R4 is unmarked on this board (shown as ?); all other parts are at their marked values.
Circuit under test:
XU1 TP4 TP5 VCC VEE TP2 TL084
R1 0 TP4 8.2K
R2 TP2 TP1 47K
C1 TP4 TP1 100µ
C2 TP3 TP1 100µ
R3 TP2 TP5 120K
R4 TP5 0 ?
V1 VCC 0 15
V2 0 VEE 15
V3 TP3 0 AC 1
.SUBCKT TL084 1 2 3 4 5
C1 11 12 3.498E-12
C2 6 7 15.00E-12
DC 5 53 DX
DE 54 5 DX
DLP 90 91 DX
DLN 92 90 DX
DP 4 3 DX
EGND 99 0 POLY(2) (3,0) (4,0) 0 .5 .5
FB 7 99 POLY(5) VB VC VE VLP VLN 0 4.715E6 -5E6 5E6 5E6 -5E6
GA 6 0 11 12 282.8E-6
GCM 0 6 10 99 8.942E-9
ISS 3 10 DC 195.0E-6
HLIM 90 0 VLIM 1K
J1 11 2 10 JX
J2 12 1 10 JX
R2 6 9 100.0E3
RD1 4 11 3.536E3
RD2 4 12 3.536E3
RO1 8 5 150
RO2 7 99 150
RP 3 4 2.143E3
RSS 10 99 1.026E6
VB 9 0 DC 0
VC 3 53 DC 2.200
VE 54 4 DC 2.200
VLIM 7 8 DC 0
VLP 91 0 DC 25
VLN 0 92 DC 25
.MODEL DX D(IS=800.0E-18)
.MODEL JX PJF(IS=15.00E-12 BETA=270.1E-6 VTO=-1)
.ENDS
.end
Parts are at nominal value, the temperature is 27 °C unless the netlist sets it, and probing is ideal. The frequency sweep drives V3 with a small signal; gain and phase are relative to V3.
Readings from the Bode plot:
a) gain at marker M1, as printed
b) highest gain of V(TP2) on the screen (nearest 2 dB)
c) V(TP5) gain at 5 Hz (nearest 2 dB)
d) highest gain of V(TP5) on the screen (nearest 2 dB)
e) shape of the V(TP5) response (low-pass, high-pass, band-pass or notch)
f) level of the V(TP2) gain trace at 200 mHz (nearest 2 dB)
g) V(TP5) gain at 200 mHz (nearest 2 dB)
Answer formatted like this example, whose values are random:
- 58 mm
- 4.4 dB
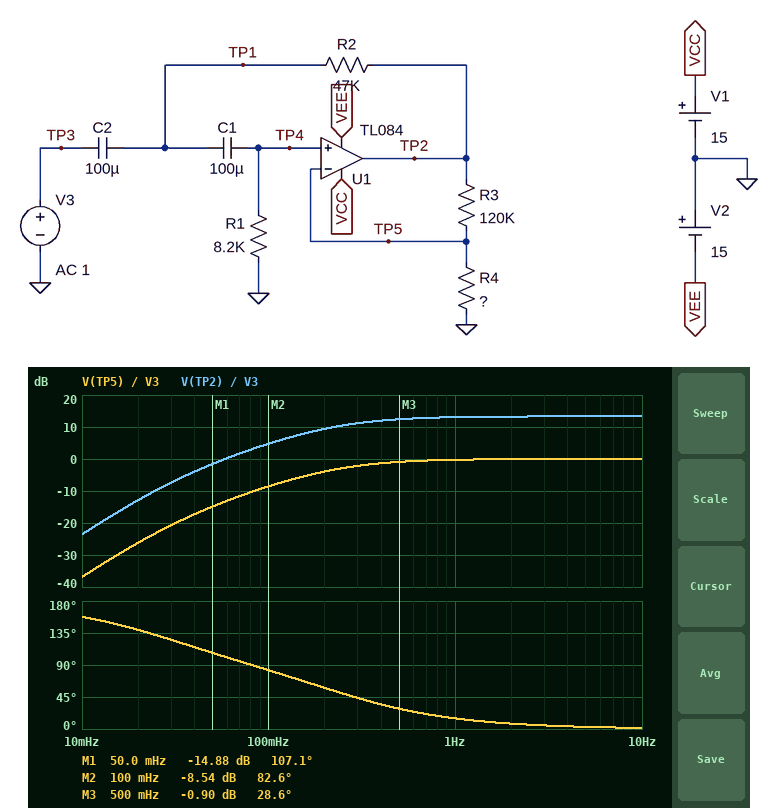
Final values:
- -14.88 dB
- 14 dB
- 0 dB
- 0 dB
- high-pass
- 10 dB
- -4 dB
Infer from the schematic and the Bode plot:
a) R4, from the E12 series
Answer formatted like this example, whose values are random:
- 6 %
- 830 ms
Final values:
- 33 kΩ
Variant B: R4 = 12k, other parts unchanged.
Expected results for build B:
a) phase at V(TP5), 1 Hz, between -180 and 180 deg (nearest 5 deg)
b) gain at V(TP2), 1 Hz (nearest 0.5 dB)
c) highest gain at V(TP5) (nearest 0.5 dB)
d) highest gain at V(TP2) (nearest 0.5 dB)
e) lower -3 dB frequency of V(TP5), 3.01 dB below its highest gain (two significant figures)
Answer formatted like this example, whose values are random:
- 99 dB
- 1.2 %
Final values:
- 5 deg
- 21.0 dB
- 4.5 dB
- 25.5 dB
- 69 mHz
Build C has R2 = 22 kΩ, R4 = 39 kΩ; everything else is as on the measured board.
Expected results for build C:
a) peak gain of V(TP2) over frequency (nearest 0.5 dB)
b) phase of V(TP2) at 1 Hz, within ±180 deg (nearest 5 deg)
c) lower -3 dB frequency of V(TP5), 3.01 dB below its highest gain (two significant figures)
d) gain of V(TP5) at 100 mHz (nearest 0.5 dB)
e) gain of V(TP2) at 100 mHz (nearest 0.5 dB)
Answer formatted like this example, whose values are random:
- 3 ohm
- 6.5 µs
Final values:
- 12.0 dB
- 10 deg
- 120 mHz
- -4.5 dB
- 7.5 dB
